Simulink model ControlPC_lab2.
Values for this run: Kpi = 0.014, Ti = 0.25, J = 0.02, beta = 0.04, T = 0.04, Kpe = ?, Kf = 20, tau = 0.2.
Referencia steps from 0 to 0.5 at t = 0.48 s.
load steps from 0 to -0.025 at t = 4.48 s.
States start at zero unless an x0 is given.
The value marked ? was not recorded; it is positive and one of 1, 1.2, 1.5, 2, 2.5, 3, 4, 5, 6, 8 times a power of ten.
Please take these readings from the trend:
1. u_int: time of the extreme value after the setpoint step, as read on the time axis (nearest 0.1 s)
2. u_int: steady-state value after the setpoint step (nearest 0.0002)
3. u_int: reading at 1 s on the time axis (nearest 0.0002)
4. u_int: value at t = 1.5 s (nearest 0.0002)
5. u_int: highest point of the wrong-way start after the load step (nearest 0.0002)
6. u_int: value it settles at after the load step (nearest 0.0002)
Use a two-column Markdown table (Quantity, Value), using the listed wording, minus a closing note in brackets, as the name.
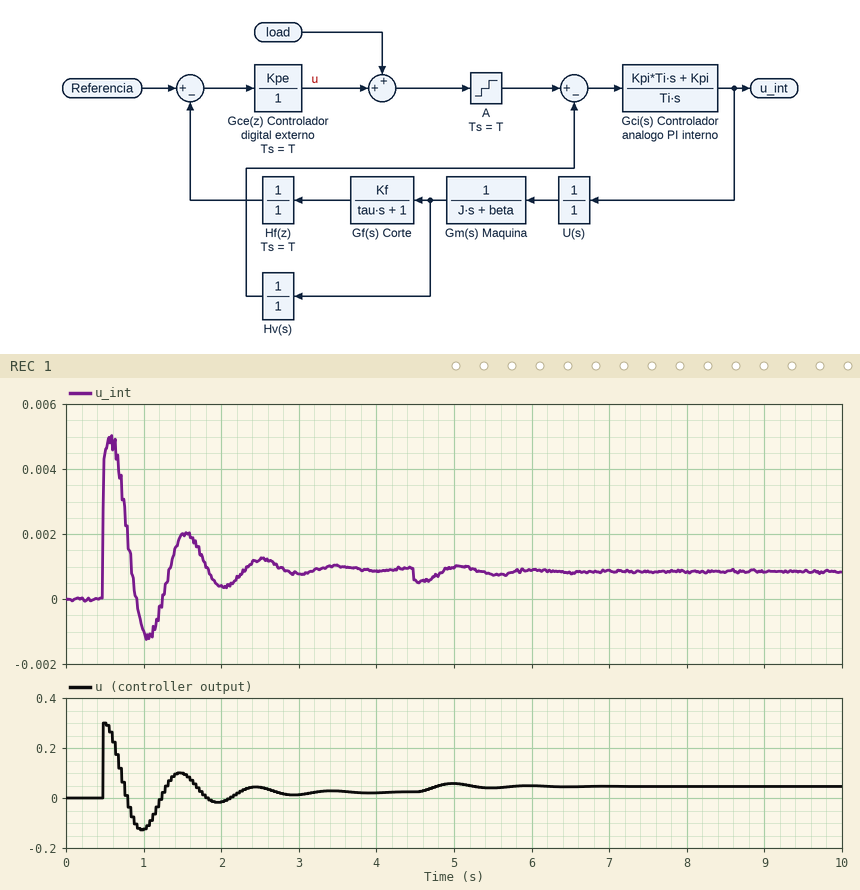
| Quantity | Value |
|---|---|
| u_int: time of the extreme value after the setpoint step, as read on the time axis | 0.6 s |
| u_int: steady-state value after the setpoint step | 0.0010 |
| u_int: reading at 1 s on the time axis | -0.0010 |
| u_int: value at t = 1.5 s | 0.0020 |
| u_int: highest point of the wrong-way start after the load step | 0.0010 |
| u_int: value it settles at after the load step | 0.0008 |
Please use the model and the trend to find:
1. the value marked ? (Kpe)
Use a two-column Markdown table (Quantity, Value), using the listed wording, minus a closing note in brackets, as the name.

| Quantity | Value |
|---|---|
| the value marked ? | 0.6 |
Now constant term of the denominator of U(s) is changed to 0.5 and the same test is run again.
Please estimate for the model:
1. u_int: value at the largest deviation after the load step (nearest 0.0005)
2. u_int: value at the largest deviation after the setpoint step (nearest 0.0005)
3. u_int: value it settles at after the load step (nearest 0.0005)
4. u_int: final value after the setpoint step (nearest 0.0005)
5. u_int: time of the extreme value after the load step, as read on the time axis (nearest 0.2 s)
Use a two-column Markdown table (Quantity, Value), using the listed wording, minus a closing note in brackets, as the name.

| Quantity | Value |
|---|---|
| u_int: value at the largest deviation after the load step | 0.0000 |
| u_int: value at the largest deviation after the setpoint step | 0.0045 |
| u_int: value it settles at after the load step | 0.0005 |
| u_int: final value after the setpoint step | 0.0005 |
| u_int: time of the extreme value after the load step, as read on the time axis | 4.6 s |
